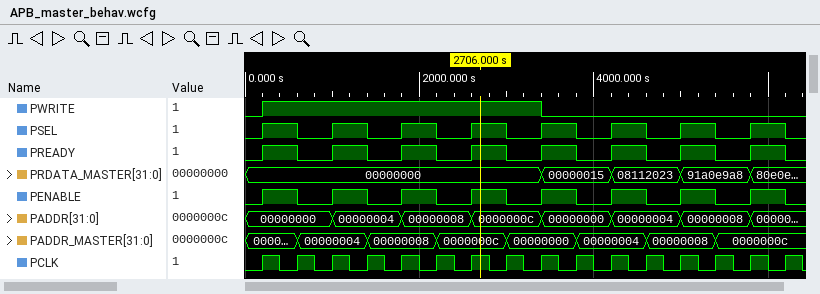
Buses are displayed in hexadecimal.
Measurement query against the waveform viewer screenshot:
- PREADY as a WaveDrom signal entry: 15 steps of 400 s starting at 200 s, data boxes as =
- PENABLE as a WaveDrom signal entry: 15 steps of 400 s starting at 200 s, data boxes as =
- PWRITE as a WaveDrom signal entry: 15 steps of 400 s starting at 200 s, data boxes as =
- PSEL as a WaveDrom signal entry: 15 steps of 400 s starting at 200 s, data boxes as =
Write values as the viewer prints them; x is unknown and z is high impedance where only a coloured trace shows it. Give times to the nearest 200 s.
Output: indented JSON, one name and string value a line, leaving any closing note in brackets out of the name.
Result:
{
  "PREADY as a WaveDrom signal entry: 15 steps of 400 s starting at 200 s, data boxes as =": "{name: 'PREADY', wave: '101010101010101'}",
  "PENABLE as a WaveDrom signal entry: 15 steps of 400 s starting at 200 s, data boxes as =": "{name: 'PENABLE', wave: '101010101010101'}",
  "PWRITE as a WaveDrom signal entry: 15 steps of 400 s starting at 200 s, data boxes as =": "{name: 'PWRITE', wave: '1.......0......'}",
  "PSEL as a WaveDrom signal entry: 15 steps of 400 s starting at 200 s, data boxes as =": "{name: 'PSEL', wave: '101010101010101'}"
}
